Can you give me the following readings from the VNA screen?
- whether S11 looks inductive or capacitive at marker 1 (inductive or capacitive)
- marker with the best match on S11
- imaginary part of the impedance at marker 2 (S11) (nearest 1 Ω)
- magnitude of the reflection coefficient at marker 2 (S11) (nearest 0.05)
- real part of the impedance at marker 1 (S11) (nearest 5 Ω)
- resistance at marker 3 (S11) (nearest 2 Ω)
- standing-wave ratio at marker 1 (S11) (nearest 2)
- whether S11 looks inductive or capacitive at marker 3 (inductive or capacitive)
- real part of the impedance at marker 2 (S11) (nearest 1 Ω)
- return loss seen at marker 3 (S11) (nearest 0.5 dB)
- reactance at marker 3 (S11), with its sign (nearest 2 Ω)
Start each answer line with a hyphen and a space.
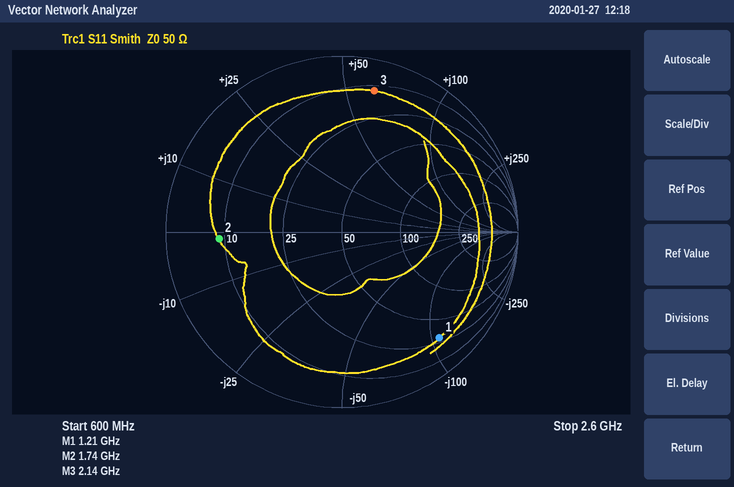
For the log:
- capacitive
- marker 2
- -1 Ω
- 0.70
- 30 Ω
- 12 Ω
- 10
- inductive
- 9 Ω
- 1.5 dB
- +62 Ω
